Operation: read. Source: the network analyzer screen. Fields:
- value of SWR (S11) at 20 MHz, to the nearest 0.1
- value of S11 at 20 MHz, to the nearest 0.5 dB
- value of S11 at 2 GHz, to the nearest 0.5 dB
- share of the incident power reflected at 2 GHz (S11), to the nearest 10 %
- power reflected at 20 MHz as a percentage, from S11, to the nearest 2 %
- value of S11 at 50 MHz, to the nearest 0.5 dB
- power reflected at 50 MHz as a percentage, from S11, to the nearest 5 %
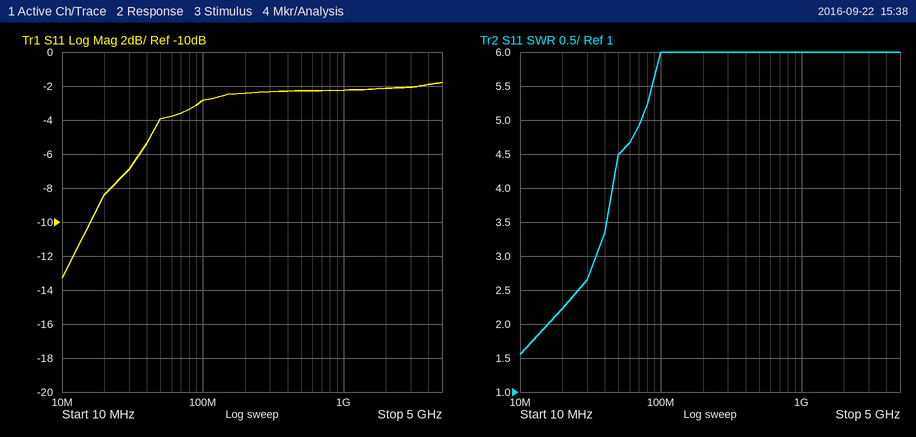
2.2
-8.5 dB
-2.0 dB
60 %
14 %
-4.0 dB
40 %
